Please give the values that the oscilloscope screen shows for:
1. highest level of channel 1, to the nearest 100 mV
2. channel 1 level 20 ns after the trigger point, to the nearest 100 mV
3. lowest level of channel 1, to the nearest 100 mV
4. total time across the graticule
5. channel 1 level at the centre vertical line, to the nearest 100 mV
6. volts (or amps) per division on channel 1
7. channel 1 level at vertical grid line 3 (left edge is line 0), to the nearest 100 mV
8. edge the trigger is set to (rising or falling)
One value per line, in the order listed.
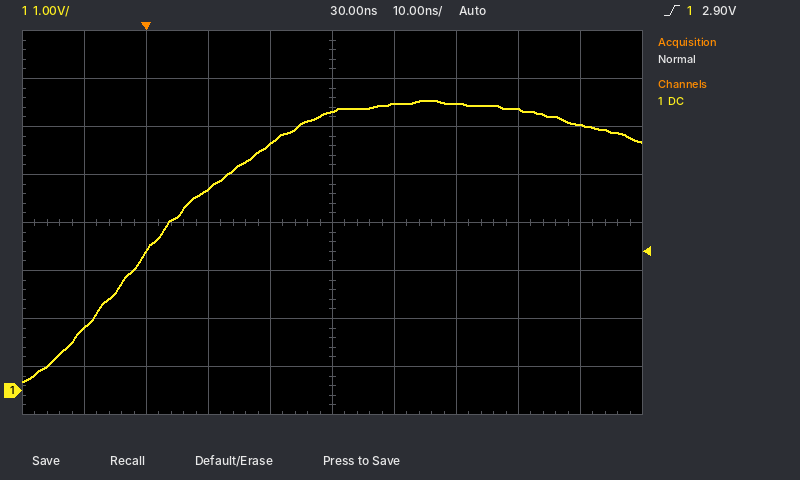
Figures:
6.0 V
5.1 V
200 mV
100 ns
5.8 V
1 V
4.2 V
rising
